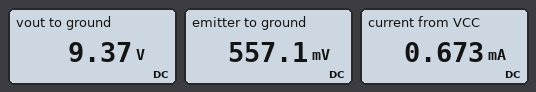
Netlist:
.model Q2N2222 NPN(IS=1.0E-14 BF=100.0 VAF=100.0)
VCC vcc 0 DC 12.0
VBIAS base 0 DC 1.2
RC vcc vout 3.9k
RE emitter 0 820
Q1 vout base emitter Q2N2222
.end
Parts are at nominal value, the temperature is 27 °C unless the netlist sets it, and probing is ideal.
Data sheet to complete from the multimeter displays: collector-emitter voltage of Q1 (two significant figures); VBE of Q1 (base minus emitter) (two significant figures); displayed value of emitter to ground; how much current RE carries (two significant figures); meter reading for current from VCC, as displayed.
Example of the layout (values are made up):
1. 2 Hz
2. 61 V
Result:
1. 8.8 V
2. 640 mV
3. 557.1 mV
4. 680 µA
5. 0.673 mA
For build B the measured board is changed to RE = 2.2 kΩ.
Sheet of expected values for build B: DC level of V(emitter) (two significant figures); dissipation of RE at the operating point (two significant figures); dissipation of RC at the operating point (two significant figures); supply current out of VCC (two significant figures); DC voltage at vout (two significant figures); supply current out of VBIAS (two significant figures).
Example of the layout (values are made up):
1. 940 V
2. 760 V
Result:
1. 580 mV
2. 150 µW
3. 270 µW
4. 260 µA
5. 11 V
6. 2.4 µA
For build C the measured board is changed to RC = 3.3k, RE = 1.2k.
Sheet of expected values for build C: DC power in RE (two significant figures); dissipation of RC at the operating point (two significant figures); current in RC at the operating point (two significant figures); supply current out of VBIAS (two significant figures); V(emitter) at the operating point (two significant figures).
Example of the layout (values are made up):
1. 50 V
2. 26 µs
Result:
1. 270 µW
2. 720 µW
3. 470 µA
4. 4.3 µA
5. 570 mV
